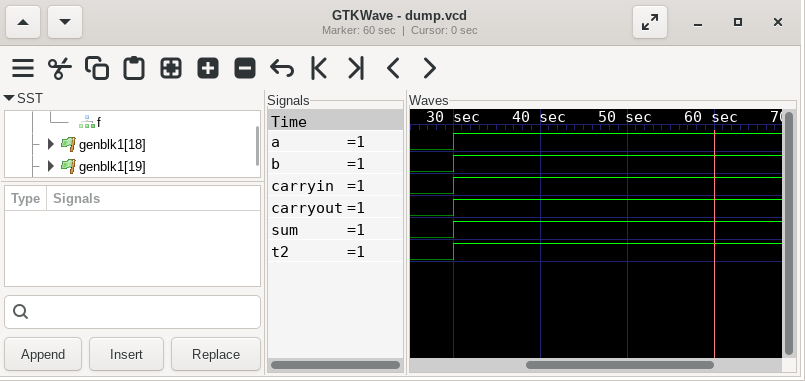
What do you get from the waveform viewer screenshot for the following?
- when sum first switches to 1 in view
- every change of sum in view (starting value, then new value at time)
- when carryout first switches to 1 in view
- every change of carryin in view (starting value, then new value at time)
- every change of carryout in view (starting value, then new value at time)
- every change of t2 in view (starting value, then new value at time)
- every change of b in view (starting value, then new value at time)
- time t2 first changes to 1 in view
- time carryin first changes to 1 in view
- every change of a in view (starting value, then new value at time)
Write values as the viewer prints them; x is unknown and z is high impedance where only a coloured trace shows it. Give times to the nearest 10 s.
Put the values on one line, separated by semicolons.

30 s; 0, 1 at 30 s; 30 s; 0, 1 at 30 s; 0, 1 at 30 s; 0, 1 at 30 s; 0, 1 at 30 s; 30 s; 30 s; 0, 1 at 30 s
